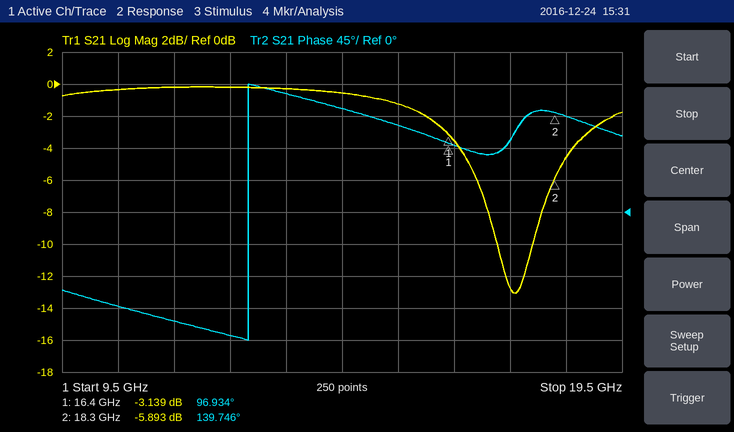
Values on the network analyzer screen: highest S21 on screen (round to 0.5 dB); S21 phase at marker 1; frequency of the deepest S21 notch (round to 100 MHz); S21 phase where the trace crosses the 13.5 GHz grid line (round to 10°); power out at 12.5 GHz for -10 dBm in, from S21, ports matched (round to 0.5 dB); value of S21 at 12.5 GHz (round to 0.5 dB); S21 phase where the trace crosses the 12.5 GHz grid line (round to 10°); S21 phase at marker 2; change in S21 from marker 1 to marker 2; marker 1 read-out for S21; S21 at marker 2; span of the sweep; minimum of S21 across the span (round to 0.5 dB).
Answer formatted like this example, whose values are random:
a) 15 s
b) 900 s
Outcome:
a) 0.0 dB
b) 96.934°
c) 17.6 GHz
d) 170°
e) -10.0 dBm
f) 0.0 dB
g) -170°
h) 139.746°
i) -2.754 dB
j) -3.139 dB
k) -5.893 dB
l) 10 GHz
m) -13.0 dB
